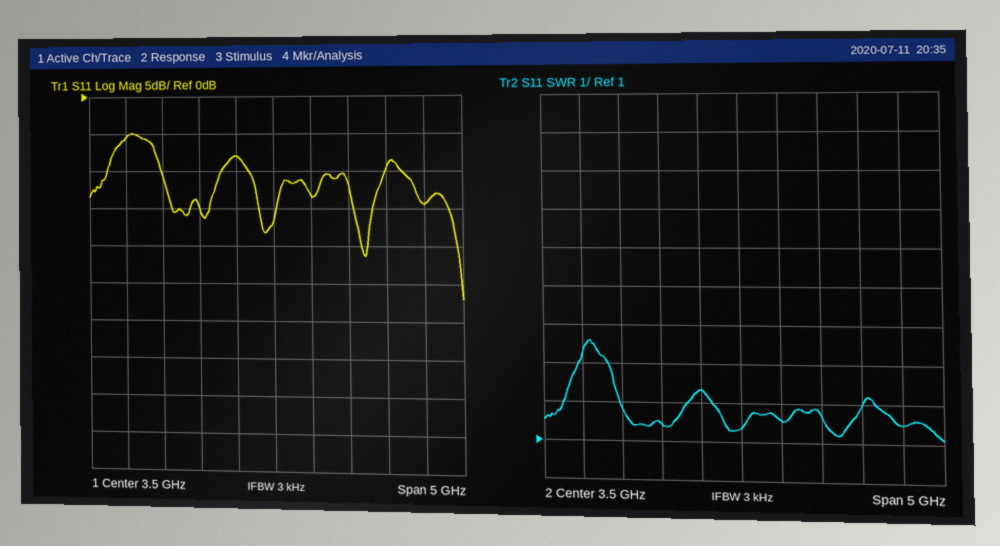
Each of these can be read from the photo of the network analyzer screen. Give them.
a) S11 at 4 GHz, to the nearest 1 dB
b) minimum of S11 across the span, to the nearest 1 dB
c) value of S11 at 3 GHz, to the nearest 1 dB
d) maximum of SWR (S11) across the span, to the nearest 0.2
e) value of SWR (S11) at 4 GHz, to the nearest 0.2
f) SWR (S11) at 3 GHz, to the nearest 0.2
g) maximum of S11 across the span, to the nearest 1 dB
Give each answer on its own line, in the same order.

-13 dB
-27 dB
-8 dB
3.6
1.6
2.4
-5 dB
